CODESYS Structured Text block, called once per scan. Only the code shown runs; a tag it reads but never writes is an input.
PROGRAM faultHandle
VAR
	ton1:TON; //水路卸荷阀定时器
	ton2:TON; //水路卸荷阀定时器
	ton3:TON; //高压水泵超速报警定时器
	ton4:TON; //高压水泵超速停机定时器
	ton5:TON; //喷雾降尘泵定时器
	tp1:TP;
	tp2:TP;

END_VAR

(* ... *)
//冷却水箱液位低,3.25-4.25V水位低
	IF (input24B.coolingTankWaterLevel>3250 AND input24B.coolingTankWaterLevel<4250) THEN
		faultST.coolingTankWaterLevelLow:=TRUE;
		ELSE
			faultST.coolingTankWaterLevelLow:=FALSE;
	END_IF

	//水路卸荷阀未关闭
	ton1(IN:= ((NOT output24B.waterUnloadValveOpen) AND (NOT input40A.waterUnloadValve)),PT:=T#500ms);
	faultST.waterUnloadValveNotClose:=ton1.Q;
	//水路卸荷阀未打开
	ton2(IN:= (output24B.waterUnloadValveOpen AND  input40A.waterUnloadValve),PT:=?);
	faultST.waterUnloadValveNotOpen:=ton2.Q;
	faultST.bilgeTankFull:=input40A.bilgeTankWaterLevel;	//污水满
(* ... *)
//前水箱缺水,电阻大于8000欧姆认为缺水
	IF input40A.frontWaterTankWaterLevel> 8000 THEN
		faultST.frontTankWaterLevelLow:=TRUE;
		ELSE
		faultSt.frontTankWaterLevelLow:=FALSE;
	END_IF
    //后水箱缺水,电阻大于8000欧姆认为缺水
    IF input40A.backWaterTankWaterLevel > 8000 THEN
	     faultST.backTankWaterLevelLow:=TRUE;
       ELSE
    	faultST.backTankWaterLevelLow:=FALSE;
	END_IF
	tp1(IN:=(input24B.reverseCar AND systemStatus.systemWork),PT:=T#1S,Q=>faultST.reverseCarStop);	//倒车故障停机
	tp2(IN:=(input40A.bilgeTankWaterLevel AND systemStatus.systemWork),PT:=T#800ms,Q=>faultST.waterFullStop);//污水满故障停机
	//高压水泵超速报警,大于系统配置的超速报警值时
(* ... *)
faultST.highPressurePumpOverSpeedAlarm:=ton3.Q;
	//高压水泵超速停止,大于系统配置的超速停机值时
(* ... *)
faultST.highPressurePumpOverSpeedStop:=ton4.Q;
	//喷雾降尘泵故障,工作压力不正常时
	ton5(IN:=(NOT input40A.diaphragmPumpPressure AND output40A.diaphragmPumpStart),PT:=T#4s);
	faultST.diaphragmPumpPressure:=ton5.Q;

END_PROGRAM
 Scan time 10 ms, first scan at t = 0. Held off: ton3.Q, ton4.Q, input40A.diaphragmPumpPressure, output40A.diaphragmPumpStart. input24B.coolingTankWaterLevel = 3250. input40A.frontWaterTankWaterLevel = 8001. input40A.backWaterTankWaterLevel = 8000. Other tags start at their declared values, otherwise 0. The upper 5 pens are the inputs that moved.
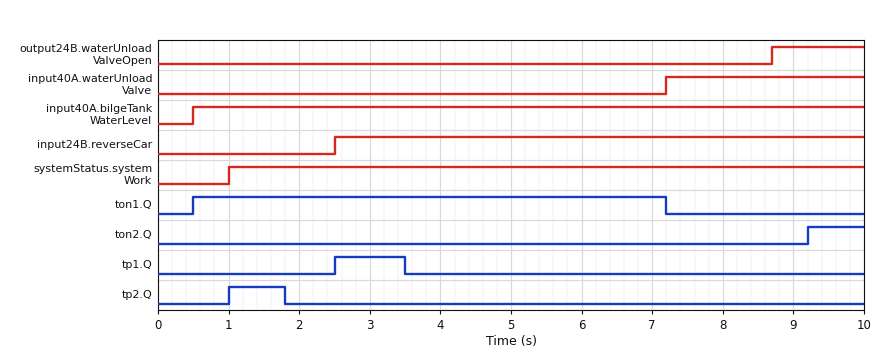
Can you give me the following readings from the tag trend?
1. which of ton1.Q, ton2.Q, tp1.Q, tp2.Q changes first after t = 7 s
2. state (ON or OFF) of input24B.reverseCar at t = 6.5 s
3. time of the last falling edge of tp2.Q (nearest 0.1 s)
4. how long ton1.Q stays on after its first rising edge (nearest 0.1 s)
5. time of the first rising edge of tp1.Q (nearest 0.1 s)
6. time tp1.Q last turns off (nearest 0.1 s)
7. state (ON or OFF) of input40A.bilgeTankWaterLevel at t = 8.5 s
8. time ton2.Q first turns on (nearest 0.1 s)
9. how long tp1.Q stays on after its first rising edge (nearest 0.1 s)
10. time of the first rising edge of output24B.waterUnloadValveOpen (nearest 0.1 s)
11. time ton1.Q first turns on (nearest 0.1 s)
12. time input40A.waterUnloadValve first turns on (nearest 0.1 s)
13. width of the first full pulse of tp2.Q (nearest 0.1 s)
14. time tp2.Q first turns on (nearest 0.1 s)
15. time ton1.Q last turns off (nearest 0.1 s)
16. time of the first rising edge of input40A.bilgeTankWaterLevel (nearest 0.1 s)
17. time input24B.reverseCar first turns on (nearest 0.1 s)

ton1.Q
ON
1.8 s
6.7 s
2.5 s
3.5 s
ON
9.2 s
1.0 s
8.7 s
0.5 s
7.2 s
0.8 s
1.0 s
7.2 s
0.5 s
2.5 s
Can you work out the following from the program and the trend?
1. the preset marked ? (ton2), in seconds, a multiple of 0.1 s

0.5 s
